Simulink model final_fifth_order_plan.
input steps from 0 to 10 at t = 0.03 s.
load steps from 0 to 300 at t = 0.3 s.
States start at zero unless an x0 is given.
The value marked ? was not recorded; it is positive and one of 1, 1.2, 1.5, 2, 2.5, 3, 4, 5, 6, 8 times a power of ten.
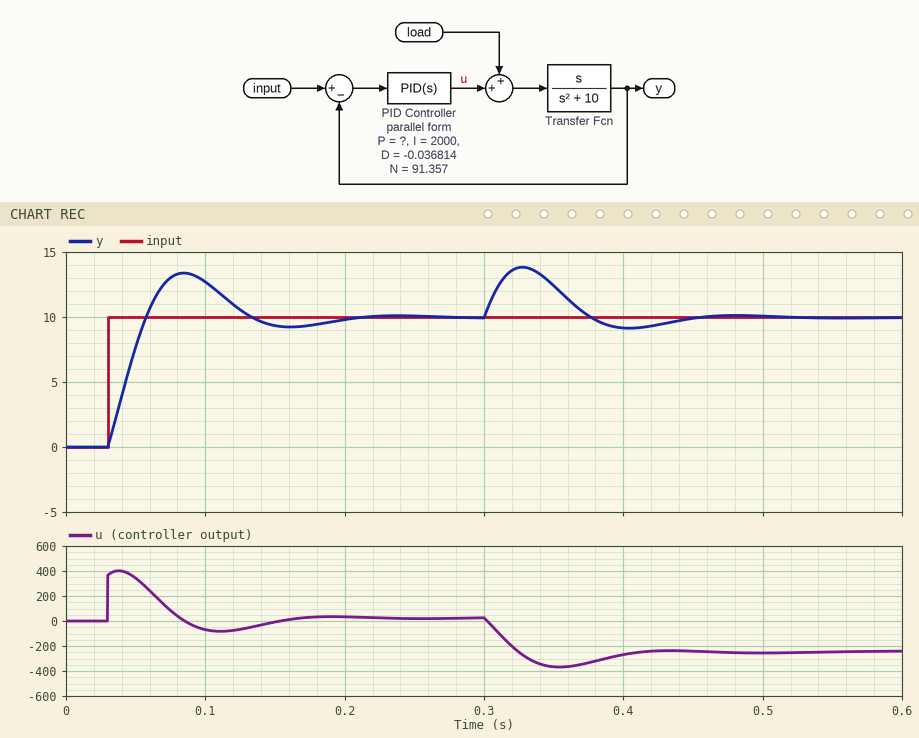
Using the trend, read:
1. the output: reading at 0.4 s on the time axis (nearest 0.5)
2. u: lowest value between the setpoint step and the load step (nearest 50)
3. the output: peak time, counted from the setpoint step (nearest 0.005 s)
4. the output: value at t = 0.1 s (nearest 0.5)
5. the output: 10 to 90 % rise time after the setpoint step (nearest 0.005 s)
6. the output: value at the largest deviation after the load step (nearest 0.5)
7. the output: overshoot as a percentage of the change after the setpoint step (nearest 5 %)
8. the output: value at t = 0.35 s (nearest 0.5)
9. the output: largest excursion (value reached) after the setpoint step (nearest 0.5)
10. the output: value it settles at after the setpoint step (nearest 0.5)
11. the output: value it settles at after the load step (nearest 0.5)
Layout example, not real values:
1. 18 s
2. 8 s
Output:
1. 9.0
2. -100
3. 0.055 s
4. 12.5
5. 0.020 s
6. 14.0
7. 35 %
8. 12.5
9. 13.5
10. 10.0
11. 10.0
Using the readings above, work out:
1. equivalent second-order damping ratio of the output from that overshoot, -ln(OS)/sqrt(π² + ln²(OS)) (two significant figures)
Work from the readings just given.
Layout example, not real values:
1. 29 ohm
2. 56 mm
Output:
1. 0.32
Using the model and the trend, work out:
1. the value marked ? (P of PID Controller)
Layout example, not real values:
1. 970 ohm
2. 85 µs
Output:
1. 40
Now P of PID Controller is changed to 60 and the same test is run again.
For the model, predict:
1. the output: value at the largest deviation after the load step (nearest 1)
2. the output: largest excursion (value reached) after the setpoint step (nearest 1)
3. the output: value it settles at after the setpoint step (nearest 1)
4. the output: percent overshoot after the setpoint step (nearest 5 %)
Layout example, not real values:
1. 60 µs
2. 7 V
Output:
1. 13
2. 12
3. 10
4. 25 %
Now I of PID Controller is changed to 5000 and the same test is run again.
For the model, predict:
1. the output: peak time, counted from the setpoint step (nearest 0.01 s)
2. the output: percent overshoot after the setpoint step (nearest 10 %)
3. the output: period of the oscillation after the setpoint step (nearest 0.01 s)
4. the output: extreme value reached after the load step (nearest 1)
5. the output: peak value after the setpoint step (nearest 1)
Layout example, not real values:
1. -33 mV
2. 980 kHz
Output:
1. 0.04 s
2. 50 %
3. 0.09 s
4. 13
5. 15
